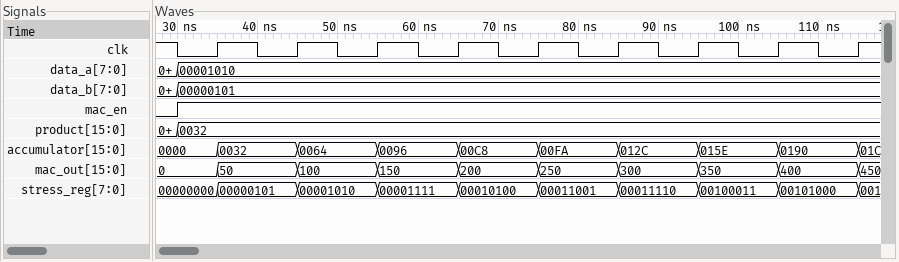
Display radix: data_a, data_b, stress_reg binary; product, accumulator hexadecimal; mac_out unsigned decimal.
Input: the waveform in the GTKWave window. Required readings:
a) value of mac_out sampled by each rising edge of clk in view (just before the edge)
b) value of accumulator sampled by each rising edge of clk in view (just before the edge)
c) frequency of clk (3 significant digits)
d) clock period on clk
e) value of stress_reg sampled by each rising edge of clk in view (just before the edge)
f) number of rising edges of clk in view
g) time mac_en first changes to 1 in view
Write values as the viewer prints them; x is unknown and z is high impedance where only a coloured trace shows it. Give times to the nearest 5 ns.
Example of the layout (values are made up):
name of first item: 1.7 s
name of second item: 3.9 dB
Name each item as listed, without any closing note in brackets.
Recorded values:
value of mac_out sampled by each rising edge of clk in view: 0, 50, 100, 150, 200, 250, 300, 350, 400
value of accumulator sampled by each rising edge of clk in view: 0000, 0032, 0064, 0096, 00C8, 00FA, 012C, 015E, 0190
frequency of clk: 100 MHz
clock period on clk: 10 ns
value of stress_reg sampled by each rising edge of clk in view: 00000000, 00000101, 00001010, 00001111, 00010100, 00011001, 00011110, 00100011, 00101000
number of rising edges of clk in view: 9
time mac_en first changes to 1 in view: 30 ns
